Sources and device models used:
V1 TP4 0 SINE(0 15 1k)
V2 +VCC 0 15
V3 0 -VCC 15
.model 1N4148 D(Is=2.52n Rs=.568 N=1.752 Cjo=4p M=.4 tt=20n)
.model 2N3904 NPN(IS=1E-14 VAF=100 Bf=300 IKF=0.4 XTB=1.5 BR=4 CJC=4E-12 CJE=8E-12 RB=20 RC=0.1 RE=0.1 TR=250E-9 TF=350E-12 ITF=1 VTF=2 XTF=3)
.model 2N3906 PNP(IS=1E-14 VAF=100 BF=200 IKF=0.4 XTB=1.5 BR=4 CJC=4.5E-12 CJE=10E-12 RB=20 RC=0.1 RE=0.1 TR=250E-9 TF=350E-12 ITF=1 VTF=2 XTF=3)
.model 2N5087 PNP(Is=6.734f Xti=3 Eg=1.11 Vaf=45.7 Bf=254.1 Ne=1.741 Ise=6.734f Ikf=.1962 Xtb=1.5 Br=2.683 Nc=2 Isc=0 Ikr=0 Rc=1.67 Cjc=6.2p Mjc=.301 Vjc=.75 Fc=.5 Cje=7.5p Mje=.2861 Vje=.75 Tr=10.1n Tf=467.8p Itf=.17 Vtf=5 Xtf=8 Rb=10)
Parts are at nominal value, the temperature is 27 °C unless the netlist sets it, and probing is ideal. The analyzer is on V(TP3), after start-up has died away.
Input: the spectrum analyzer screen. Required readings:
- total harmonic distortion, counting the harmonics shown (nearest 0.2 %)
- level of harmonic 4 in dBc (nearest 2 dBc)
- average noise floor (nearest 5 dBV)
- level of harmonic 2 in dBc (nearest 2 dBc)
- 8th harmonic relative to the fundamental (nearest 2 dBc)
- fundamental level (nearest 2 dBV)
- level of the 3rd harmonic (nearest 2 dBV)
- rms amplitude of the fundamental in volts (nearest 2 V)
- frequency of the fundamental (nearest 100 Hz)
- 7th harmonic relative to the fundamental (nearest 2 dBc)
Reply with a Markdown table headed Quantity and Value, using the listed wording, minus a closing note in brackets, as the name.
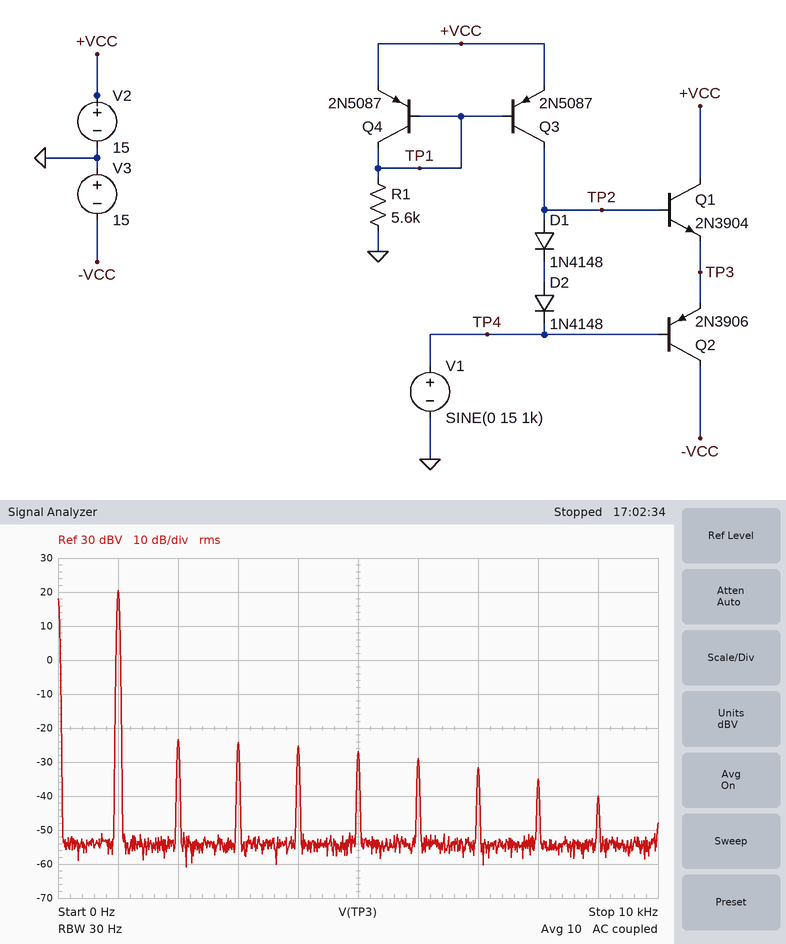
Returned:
| Quantity | Value |
|---|---|
| total harmonic distortion, counting the harmonics shown | 1.2 % |
| level of harmonic 4 in dBc | -46 dBc |
| average noise floor | -55 dBV |
| level of harmonic 2 in dBc | -44 dBc |
| 8th harmonic relative to the fundamental | -56 dBc |
| fundamental level | 20 dBV |
| level of the 3rd harmonic | -24 dBV |
| rms amplitude of the fundamental in volts | 10 V |
| frequency of the fundamental | 1.0 kHz |
| 7th harmonic relative to the fundamental | -52 dBc |
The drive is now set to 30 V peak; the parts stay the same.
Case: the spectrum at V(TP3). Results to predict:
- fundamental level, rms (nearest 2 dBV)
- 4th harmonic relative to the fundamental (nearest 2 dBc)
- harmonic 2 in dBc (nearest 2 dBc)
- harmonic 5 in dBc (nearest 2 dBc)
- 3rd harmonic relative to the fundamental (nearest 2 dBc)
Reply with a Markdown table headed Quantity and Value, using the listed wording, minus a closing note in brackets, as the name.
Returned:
| Quantity | Value |
|---|---|
| fundamental level, rms | 24 dBV |
| 4th harmonic relative to the fundamental | -34 dBc |
| harmonic 2 in dBc | -20 dBc |
| harmonic 5 in dBc | -32 dBc |
| 3rd harmonic relative to the fundamental | -18 dBc |
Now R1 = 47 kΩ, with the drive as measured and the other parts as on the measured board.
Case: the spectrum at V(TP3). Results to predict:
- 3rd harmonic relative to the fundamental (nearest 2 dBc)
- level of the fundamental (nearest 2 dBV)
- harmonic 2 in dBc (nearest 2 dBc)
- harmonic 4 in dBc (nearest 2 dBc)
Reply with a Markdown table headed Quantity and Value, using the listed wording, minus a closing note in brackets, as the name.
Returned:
| Quantity | Value |
|---|---|
| 3rd harmonic relative to the fundamental | -46 dBc |
| level of the fundamental | 20 dBV |
| harmonic 2 in dBc | -46 dBc |
| harmonic 4 in dBc | -48 dBc |
